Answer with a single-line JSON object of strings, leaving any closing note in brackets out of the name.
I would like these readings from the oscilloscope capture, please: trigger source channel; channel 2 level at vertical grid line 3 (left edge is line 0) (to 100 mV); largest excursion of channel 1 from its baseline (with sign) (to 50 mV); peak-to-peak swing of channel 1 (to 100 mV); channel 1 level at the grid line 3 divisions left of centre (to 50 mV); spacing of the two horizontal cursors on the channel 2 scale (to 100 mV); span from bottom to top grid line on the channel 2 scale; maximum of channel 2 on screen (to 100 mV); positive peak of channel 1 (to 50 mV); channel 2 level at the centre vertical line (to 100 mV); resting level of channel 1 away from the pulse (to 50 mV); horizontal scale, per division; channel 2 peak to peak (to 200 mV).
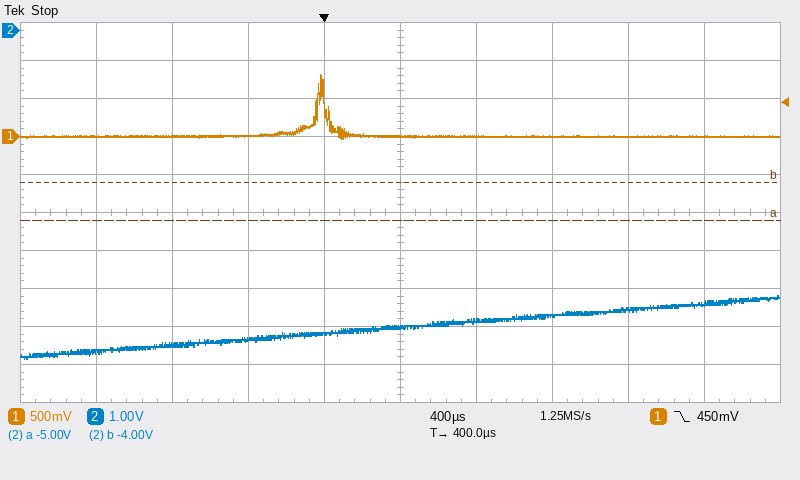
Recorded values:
{"trigger source channel": "channel 1", "channel 2 level at vertical grid line 3 (left edge is line 0)": "-8.1 V", "largest excursion of channel 1 from its baseline (with sign)": "+800 mV", "peak-to-peak swing of channel 1": "800 mV", "channel 1 level at the grid line 3 divisions left of centre": "0 mV", "spacing of the two horizontal cursors on the channel 2 scale": "1.0 V", "span from bottom to top grid line on the channel 2 scale": "10 V", "maximum of channel 2 on screen": "-7.0 V", "positive peak of channel 1": "800 mV", "channel 2 level at the centre vertical line": "-7.8 V", "resting level of channel 1 away from the pulse": "0 mV", "horizontal scale, per division": "400 µs", "channel 2 peak to peak": "1.6 V"}
